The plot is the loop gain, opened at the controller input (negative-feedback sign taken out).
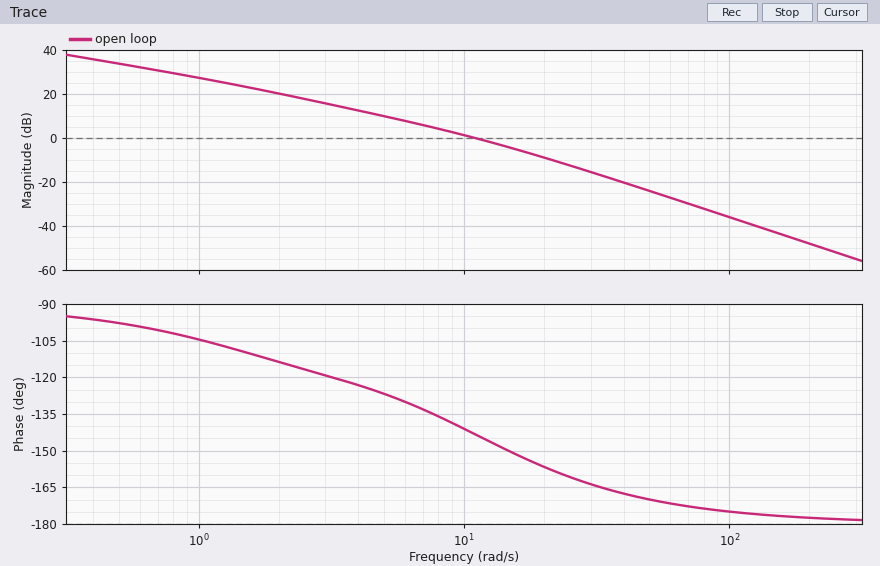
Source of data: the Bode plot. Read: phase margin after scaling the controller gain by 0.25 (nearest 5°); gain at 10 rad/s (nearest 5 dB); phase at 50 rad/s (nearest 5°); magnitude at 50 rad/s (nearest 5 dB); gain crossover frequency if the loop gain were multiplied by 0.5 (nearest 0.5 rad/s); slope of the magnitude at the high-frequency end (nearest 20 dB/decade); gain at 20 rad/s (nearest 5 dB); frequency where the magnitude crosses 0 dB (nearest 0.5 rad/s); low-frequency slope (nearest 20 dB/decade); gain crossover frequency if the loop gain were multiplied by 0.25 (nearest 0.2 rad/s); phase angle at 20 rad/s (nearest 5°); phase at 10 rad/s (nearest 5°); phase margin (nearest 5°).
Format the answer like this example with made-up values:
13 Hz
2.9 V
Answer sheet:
55°
0 dB
-170°
-25 dB
7.0 rad/s
-40 dB/decade
-10 dB
11.0 rad/s
-20 dB/decade
4.2 rad/s
-155°
-140°
35°
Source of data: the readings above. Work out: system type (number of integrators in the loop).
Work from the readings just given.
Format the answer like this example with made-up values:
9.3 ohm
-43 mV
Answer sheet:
1
